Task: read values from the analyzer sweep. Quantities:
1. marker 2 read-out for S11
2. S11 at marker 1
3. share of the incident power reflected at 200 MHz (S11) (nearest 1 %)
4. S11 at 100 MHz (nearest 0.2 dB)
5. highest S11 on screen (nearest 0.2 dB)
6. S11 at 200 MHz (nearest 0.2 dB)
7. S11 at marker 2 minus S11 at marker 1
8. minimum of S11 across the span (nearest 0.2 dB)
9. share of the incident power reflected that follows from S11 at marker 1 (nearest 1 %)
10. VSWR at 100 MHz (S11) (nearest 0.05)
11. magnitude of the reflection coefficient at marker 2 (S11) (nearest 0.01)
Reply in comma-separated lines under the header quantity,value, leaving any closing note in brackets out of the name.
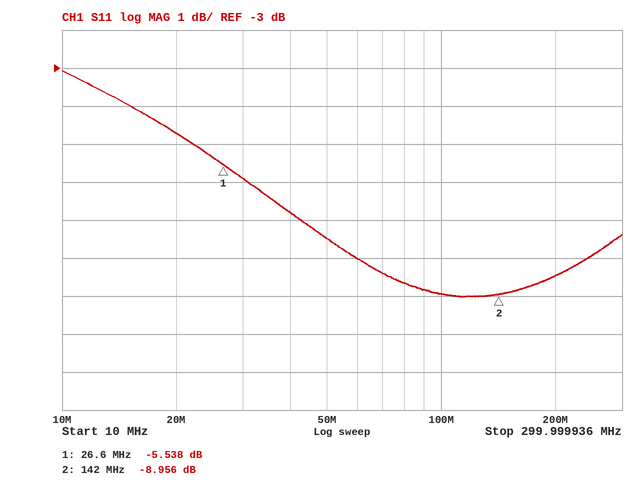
quantity,value
marker 2 read-out for S11,-8.956 dB
S11 at marker 1,-5.538 dB
share of the incident power reflected at 200 MHz (S11),14 %
S11 at 100 MHz,-9.0 dB
highest S11 on screen,-3.0 dB
S11 at 200 MHz,-8.4 dB
S11 at marker 2 minus S11 at marker 1,-3.418 dB
minimum of S11 across the span,-9.0 dB
share of the incident power reflected that follows from S11 at marker 1,28 %
VSWR at 100 MHz (S11),2.10
magnitude of the reflection coefficient at marker 2 (S11),0.36
